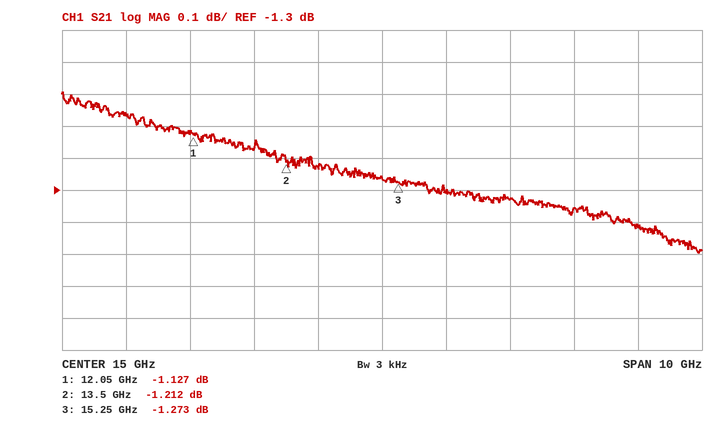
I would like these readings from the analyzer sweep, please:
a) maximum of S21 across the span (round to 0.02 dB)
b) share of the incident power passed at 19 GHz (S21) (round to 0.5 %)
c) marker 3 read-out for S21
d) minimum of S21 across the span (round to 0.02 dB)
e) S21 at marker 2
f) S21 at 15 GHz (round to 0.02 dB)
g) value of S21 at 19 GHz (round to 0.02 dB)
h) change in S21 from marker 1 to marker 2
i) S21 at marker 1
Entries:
-1.00 dB
72.0 %
-1.273 dB
-1.50 dB
-1.212 dB
-1.26 dB
-1.42 dB
-0.085 dB
-1.127 dB
